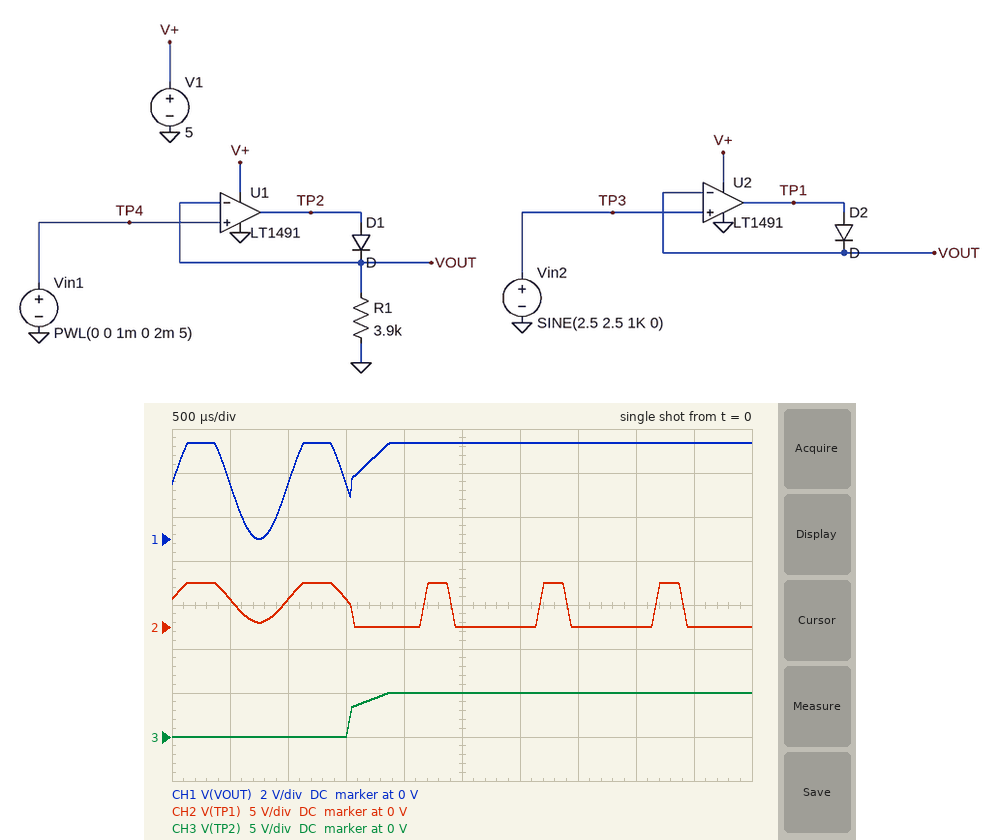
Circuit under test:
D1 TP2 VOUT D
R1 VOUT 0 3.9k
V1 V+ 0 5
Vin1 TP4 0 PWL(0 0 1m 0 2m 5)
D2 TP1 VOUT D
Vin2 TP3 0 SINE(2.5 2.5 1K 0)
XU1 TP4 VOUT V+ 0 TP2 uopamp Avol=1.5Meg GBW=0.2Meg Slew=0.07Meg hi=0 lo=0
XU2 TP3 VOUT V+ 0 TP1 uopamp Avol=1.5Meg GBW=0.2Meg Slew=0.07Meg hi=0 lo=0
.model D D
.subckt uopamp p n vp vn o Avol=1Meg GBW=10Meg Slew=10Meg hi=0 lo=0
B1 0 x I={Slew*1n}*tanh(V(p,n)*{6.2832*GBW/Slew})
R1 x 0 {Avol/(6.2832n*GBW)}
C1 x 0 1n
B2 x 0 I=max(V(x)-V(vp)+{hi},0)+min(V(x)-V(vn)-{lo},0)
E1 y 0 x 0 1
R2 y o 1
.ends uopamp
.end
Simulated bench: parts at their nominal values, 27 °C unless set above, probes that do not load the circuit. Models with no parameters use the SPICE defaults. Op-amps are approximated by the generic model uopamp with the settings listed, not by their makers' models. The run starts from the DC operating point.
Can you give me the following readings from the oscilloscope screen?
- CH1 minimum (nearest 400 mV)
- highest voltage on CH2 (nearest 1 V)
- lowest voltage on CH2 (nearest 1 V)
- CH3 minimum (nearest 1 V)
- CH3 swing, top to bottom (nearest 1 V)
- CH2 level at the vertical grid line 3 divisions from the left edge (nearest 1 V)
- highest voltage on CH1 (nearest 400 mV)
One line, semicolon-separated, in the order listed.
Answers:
0 V; 5 V; 0 V; 0 V; 5 V; 3 V; 4.4 V
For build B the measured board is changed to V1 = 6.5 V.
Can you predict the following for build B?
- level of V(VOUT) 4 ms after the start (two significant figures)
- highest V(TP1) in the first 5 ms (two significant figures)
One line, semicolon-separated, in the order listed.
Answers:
5.0 V; 5.7 V
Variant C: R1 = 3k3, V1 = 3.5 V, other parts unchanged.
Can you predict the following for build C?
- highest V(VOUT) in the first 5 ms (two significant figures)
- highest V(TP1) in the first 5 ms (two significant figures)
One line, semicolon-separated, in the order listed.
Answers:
2.9 V; 3.5 V
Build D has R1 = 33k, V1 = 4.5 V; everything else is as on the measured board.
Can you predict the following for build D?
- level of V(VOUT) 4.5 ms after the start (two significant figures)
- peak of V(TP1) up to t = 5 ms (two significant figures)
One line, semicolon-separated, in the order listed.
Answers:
3.9 V; 4.5 V
